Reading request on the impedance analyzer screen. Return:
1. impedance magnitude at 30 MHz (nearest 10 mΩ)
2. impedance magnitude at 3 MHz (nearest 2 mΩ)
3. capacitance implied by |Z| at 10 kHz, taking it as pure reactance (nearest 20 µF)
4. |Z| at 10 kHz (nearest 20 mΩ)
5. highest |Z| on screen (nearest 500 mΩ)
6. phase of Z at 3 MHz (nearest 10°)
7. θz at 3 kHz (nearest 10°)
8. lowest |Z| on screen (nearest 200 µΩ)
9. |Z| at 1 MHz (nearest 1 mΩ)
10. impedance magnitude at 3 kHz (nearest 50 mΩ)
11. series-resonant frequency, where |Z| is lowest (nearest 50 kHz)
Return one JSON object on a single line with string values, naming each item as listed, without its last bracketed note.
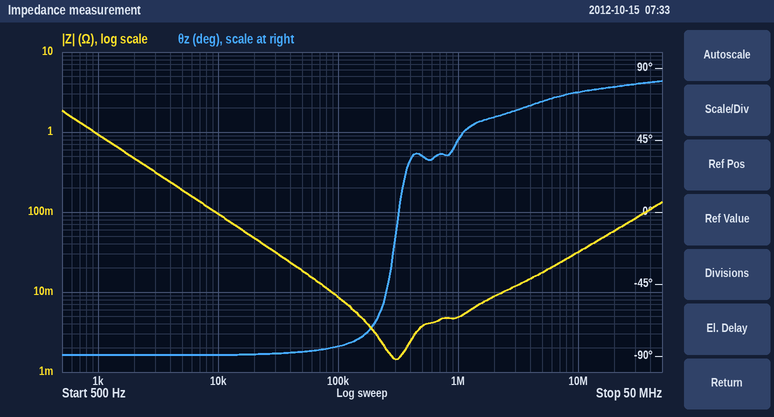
{"impedance magnitude at 30 MHz": "80 mΩ", "impedance magnitude at 3 MHz": "12 mΩ", "capacitance implied by |Z| at 10 kHz, taking it as pure reactance": "160 µF", "|Z| at 10 kHz": "100 mΩ", "highest |Z| on screen": "2.0 Ω", "phase of Z at 3 MHz": "60°", "θz at 3 kHz": "-90°", "lowest |Z| on screen": "1.4 mΩ", "|Z| at 1 MHz": "5 mΩ", "impedance magnitude at 3 kHz": "300 mΩ", "series-resonant frequency, where |Z| is lowest": "300 kHz"}
